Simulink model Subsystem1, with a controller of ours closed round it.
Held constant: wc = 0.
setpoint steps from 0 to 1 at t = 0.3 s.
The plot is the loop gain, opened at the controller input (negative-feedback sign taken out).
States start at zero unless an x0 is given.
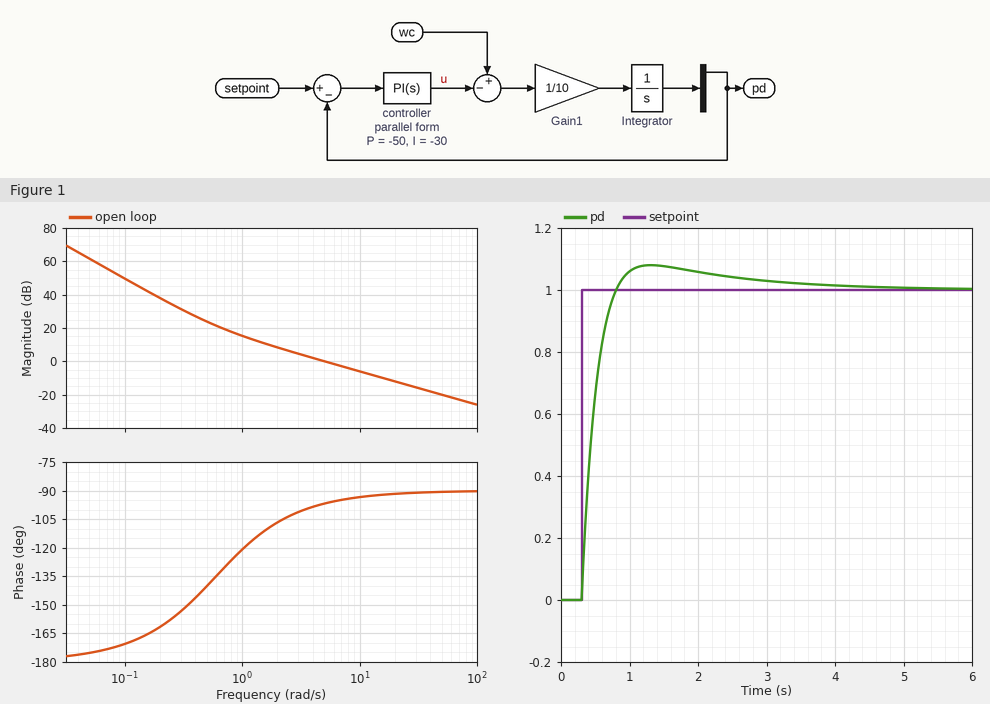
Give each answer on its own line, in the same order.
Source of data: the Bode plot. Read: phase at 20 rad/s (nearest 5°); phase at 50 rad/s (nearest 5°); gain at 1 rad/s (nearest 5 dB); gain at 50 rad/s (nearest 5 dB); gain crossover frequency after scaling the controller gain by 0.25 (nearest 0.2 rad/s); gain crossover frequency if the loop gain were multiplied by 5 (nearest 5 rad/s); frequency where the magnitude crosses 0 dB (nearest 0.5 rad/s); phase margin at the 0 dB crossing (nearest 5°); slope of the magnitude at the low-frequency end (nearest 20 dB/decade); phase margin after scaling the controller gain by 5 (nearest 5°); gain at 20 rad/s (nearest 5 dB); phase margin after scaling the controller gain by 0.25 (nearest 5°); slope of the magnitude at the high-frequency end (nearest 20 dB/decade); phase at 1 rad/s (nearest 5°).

-90°
-90°
15 dB
-20 dB
1.4 rad/s
25 rad/s
5.0 rad/s
85°
-40 dB/decade
90°
-10 dB
65°
-20 dB/decade
-120°
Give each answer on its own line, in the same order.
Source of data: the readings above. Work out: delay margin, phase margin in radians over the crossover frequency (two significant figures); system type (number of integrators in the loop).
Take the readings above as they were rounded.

0.30 s
2
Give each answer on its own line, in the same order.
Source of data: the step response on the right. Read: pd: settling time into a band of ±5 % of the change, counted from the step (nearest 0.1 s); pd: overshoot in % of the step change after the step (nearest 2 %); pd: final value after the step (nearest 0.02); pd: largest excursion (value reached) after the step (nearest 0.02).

1.9 s
8 %
1.00
1.08
